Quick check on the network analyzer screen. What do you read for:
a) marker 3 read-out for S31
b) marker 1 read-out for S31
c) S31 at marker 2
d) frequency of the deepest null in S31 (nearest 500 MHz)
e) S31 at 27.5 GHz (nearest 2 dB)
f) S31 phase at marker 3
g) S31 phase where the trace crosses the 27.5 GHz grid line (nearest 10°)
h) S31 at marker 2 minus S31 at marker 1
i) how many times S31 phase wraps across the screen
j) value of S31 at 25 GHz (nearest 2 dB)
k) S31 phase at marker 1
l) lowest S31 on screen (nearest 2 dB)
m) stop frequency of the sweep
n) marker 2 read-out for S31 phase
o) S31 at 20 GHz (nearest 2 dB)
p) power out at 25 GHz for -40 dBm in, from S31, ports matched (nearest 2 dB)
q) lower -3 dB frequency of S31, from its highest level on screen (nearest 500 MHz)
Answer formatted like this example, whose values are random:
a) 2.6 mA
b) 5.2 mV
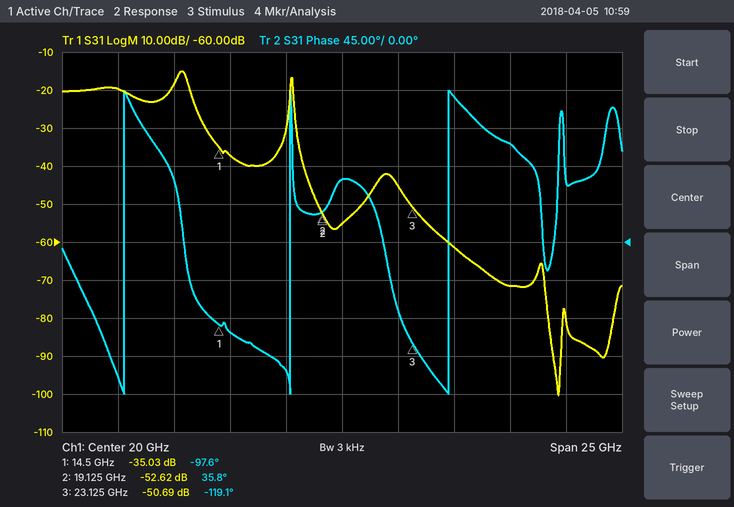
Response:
a) -50.69 dB
b) -35.03 dB
c) -52.62 dB
d) 29.5 GHz
e) -72 dB
f) -119.1°
g) 120°
h) -17.59 dB
i) 3
j) -62 dB
k) -97.6°
l) -100 dB
m) 32.5 GHz
n) 35.8°
o) -56 dB
p) -102 dBm
q) 12.5 GHz
